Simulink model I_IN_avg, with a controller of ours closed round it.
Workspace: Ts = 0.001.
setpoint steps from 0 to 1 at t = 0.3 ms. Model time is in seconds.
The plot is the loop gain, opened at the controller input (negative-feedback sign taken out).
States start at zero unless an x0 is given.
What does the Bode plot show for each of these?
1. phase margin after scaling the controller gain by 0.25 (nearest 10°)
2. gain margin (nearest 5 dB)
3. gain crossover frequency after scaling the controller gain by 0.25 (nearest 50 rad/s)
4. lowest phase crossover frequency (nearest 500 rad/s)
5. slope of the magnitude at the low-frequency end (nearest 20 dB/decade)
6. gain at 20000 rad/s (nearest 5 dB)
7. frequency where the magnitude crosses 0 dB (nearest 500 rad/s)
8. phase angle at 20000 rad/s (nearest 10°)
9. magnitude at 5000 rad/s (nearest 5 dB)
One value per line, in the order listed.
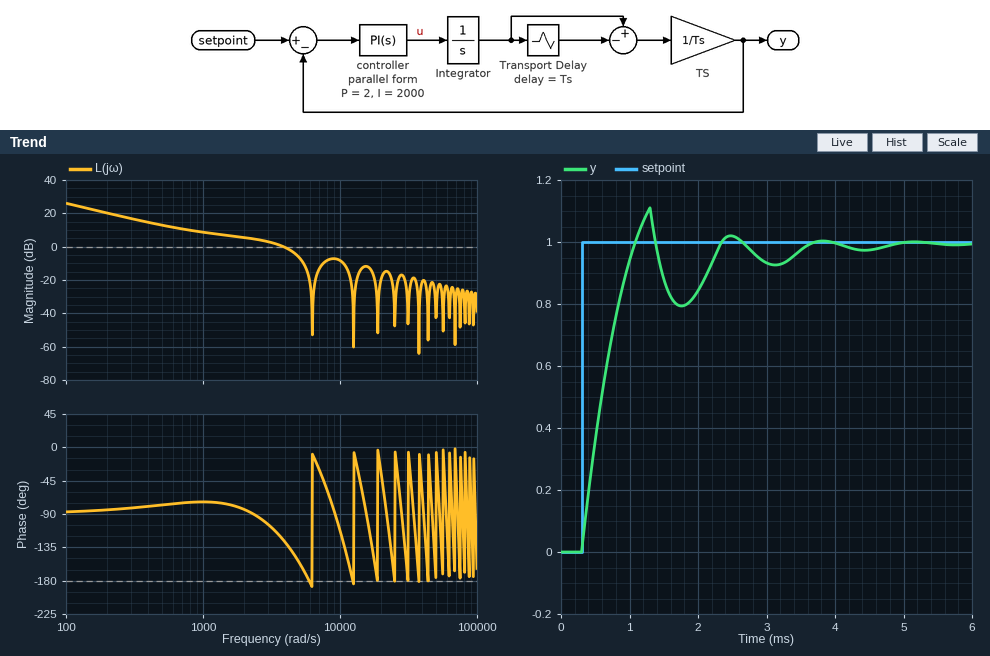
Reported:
100°
20 dB
550 rad/s
6000 rad/s
-20 dB/decade
-20 dB
4000 rad/s
-40°
-5 dB
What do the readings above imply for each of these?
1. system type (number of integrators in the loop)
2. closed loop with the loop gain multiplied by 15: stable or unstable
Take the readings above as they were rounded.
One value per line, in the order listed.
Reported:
1
unstable
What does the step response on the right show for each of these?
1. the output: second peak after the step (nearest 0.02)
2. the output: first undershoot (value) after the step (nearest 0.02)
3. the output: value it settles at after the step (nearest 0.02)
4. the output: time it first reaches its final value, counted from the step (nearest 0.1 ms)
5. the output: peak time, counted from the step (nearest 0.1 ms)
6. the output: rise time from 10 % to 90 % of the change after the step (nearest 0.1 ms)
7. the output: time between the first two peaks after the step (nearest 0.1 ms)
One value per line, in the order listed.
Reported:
1.02
0.80
1.00
0.8 ms
1.0 ms
0.6 ms
1.2 ms
